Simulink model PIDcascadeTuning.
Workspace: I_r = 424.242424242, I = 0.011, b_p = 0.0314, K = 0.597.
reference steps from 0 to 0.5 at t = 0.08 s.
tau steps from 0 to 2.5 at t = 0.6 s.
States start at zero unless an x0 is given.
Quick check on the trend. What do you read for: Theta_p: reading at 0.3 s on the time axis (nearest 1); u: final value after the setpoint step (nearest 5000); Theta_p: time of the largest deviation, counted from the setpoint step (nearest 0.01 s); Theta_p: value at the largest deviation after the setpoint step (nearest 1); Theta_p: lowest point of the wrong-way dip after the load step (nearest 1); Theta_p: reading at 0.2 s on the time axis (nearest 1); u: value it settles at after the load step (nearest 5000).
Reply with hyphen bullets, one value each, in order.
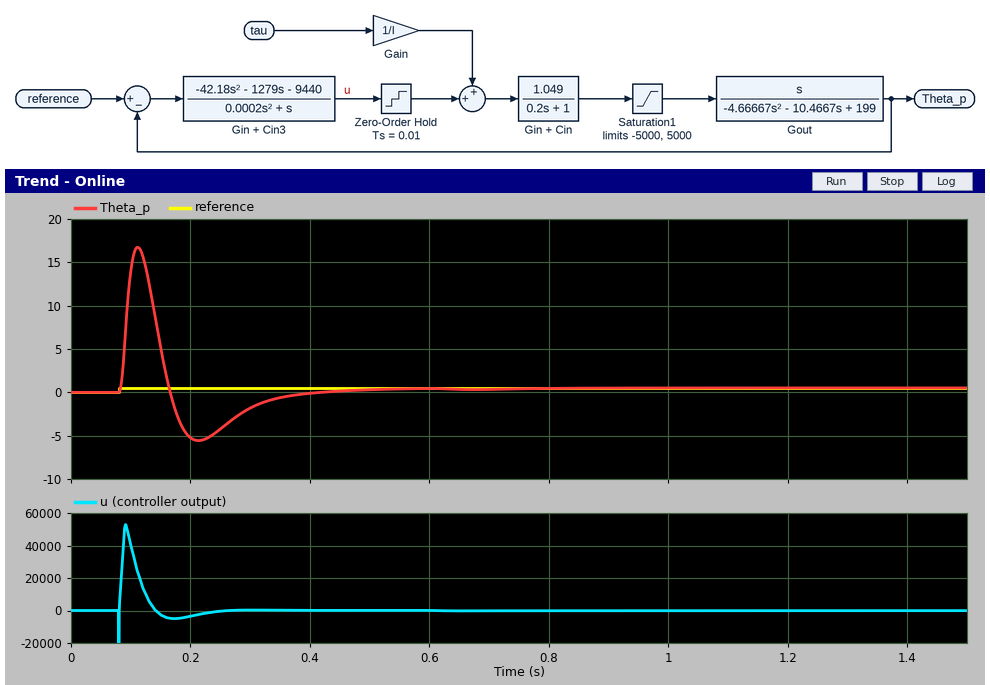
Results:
- -2
- 0
- 0.03 s
- 17
- 0
- -5
- 0
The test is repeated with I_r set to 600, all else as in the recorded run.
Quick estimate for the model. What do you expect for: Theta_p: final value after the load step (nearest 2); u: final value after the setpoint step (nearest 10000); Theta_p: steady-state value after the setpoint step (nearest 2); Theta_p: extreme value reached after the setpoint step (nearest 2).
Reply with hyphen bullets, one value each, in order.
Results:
- 0
- 0
- 0
- 14
